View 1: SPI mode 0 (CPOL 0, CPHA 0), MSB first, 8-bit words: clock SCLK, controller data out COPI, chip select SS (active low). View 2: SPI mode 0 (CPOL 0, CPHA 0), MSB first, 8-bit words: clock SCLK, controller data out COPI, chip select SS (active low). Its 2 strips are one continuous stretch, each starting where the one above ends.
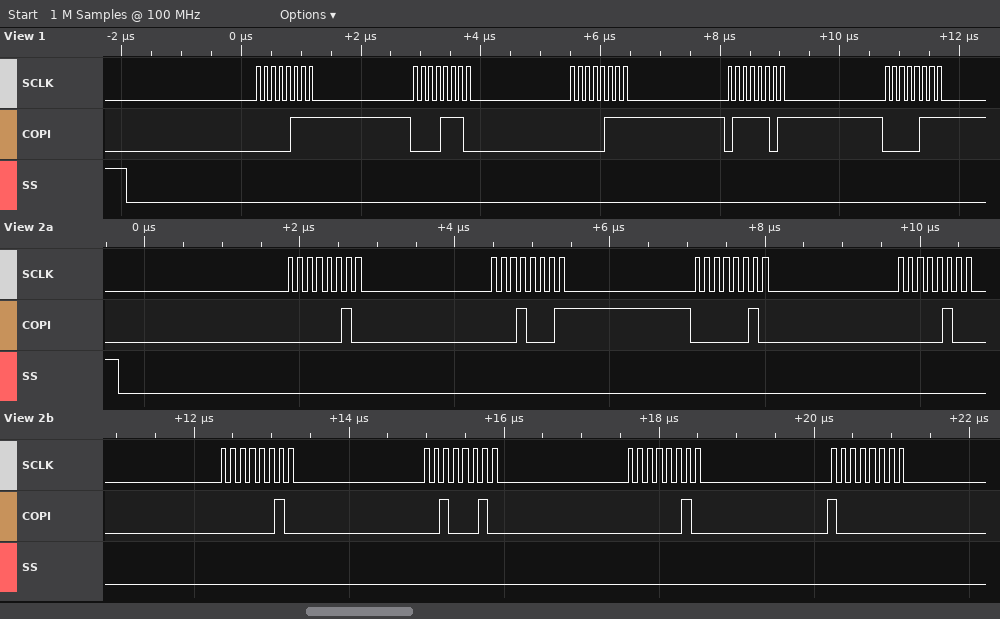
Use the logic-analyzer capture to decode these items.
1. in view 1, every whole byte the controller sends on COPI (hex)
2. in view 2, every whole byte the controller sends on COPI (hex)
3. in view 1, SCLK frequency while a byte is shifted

07 0E 07 7D 07
02 11 02 04 02 22 02 80
8 MHz
